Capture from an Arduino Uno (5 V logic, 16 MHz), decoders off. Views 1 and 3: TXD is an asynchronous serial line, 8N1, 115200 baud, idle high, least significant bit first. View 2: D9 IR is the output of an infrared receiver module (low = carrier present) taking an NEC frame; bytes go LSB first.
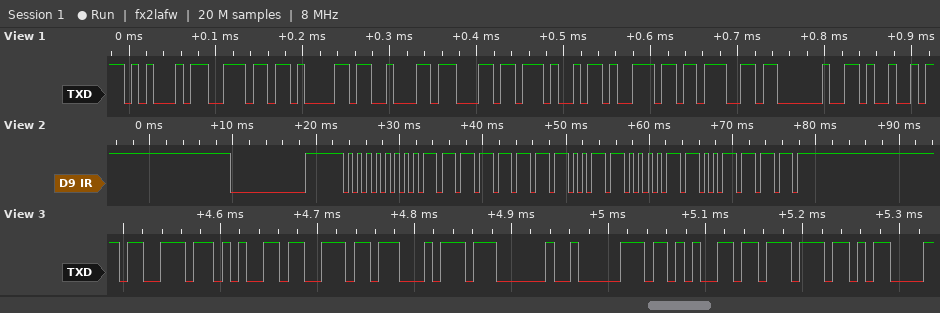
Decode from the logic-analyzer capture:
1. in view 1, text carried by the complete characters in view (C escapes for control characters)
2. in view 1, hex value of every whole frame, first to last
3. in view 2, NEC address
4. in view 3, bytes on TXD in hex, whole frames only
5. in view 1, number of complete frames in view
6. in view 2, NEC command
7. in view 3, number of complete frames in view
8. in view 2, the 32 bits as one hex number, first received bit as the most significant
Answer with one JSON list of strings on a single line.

["\"Enabling I\"", "0x45 0x6E 0x61 0x62 0x6C 0x69 0x6E 0x67 0x20 0x49", "0x00", "73 65 6E 74 20 70 65 77 0D", "10", "0x0C", "9", "0x00FF30CF"]
